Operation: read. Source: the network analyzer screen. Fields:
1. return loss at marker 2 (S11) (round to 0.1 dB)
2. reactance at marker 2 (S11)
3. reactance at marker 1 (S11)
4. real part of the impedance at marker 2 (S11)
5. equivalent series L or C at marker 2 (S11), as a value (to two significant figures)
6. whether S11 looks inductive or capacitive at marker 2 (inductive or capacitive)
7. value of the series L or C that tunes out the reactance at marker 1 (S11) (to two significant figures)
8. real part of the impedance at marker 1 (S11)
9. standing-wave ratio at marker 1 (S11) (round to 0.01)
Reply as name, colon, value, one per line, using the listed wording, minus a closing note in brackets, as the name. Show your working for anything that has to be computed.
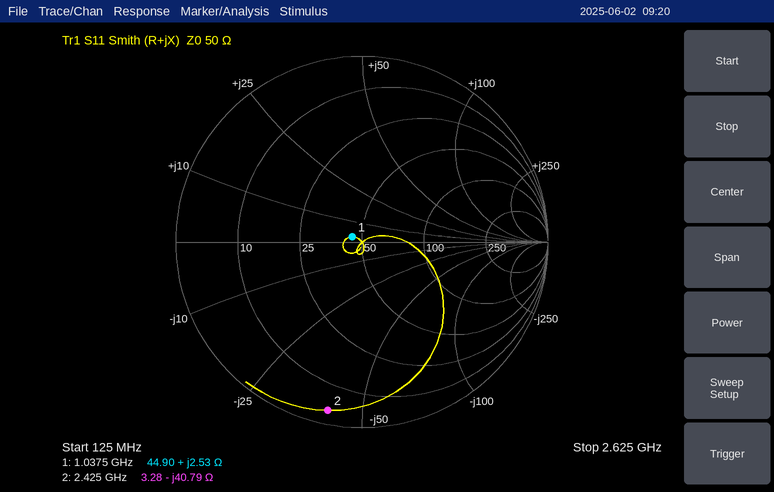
return loss at marker 2 (S11): 0.7 dB
reactance at marker 2: -40.79 Ω
reactance at marker 1: +2.53 Ω
real part of the impedance at marker 2: 3.28 Ω
equivalent series L or C at marker 2 (S11), as a value: C = 1/(2π × 2.425 GHz × 40.79 Ω) ≈ 1.6 pF
whether S11 looks inductive or capacitive at marker 2: capacitive
value of the series L or C that tunes out the reactance at marker 1 (S11): C = 1/(2π × 1.0375 GHz × 2.53 Ω) ≈ 61 pF
real part of the impedance at marker 1: 44.90 Ω
standing-wave ratio at marker 1 (S11): 1.13
